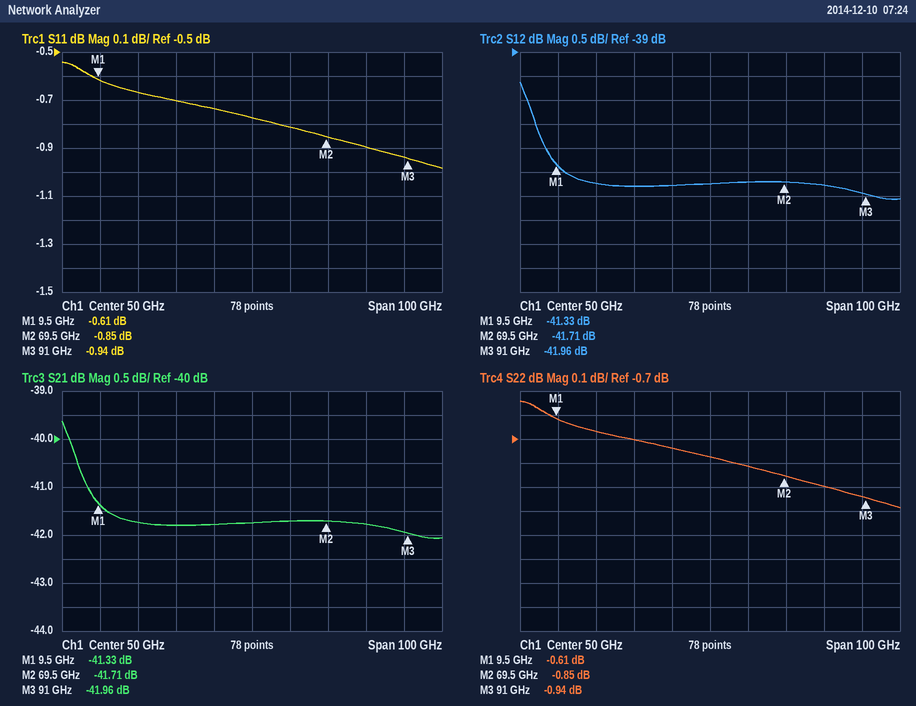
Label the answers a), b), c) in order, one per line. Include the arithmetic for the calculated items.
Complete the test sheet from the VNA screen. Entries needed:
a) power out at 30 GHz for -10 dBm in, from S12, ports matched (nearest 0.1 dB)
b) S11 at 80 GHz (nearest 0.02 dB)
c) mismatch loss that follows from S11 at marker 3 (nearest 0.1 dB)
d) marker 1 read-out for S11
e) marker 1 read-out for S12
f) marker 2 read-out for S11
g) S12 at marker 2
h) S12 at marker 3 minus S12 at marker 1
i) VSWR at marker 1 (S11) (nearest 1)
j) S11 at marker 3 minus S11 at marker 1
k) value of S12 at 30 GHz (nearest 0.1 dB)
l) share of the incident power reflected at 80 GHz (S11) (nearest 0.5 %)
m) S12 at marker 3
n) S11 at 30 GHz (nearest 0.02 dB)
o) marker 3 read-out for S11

a) -10 dBm + (-41.8 dB) = -51.8 dBm
b) -0.90 dB
c) −10 log10(1 − 10^(-0.94/10)) ≈ 7.1 dB
d) -0.61 dB
e) -41.33 dB
f) -0.85 dB
g) -41.71 dB
h) -41.96 − (-41.33) = -0.63 dB
i) (1 + 0.9322)/(1 − 0.9322) ≈ 28
j) -0.94 − (-0.61) = -0.33 dB
k) -41.8 dB
l) 10^(-0.9/10) ≈ 81.3 %, so 81.5 % to the nearest 0.5 %
m) -41.96 dB
n) -0.70 dB
o) -0.94 dB
